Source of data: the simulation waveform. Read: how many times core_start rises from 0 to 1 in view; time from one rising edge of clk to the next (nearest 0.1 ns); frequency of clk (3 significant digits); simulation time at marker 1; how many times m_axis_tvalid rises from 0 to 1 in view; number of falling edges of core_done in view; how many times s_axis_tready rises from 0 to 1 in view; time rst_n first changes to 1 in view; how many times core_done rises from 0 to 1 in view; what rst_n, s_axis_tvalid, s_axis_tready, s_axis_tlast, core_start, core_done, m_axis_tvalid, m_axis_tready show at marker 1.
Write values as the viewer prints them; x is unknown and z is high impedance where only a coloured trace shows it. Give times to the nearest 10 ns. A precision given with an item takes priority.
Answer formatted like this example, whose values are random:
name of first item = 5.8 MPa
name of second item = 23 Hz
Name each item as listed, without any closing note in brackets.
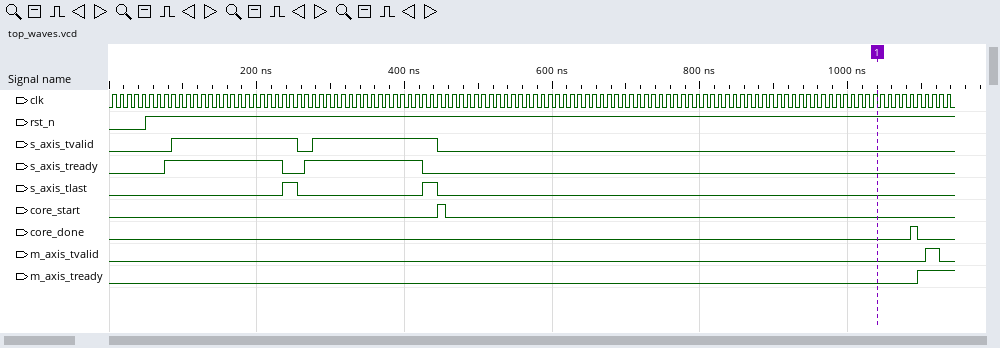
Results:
how many times core_start rises from 0 to 1 in view = 1
time from one rising edge of clk to the next = 10 ns
frequency of clk = 100 MHz
simulation time at marker 1 = 1040 ns
how many times m_axis_tvalid rises from 0 to 1 in view = 1
number of falling edges of core_done in view = 1
how many times s_axis_tready rises from 0 to 1 in view = 2
time rst_n first changes to 1 in view = 50 ns
how many times core_done rises from 0 to 1 in view = 1
what rst_n, s_axis_tvalid, s_axis_tready, s_axis_tlast, core_start, core_done, m_axis_tvalid, m_axis_tready show at marker 1 = rst_n=1, s_axis_tvalid=0, s_axis_tready=0, s_axis_tlast=0, core_start=0, core_done=0, m_axis_tvalid=0, m_axis_tready=0
